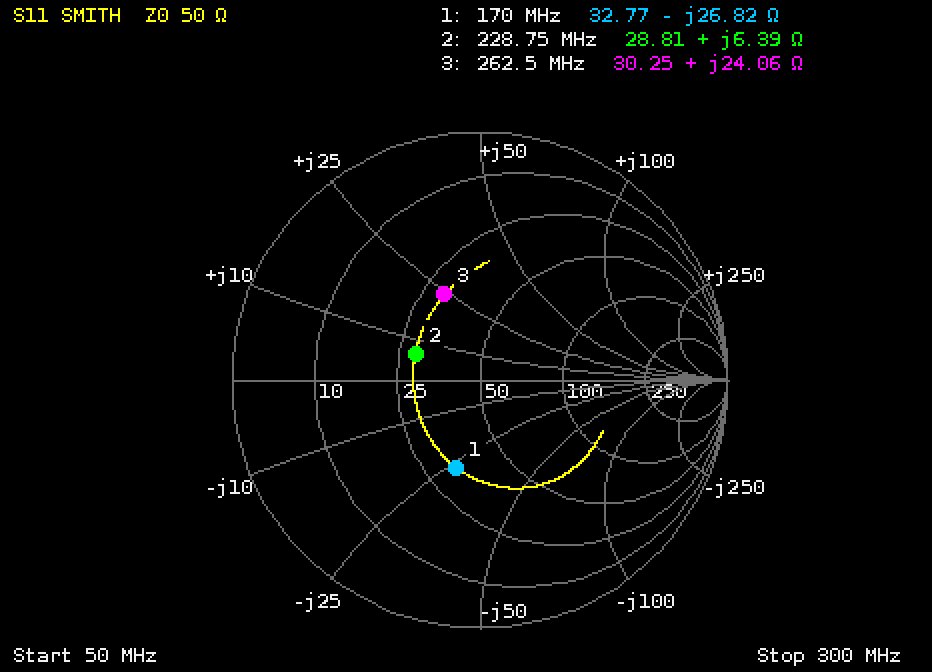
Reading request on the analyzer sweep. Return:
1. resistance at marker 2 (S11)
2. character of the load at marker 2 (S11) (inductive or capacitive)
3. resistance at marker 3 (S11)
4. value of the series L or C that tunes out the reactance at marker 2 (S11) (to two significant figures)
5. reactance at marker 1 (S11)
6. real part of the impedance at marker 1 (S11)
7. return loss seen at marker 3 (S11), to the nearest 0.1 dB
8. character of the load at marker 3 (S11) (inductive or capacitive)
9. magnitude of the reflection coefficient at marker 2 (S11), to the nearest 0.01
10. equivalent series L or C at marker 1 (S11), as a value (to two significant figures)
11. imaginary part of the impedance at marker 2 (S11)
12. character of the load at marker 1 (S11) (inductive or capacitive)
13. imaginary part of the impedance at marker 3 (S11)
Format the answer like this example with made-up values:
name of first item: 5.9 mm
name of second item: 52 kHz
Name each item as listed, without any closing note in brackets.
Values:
resistance at marker 2: 28.81 Ω
character of the load at marker 2 (S11): inductive
resistance at marker 3: 30.25 Ω
value of the series L or C that tunes out the reactance at marker 2 (S11): 110 pF
reactance at marker 1: -26.82 Ω
real part of the impedance at marker 1: 32.77 Ω
return loss seen at marker 3 (S11), to the nearest 0.1 dB: 8.6 dB
character of the load at marker 3 (S11): inductive
magnitude of the reflection coefficient at marker 2 (S11), to the nearest 0.01: 0.28
equivalent series L or C at marker 1 (S11), as a value: 35 pF
imaginary part of the impedance at marker 2: +6.39 Ω
character of the load at marker 1 (S11): capacitive
imaginary part of the impedance at marker 3: +24.06 Ω
